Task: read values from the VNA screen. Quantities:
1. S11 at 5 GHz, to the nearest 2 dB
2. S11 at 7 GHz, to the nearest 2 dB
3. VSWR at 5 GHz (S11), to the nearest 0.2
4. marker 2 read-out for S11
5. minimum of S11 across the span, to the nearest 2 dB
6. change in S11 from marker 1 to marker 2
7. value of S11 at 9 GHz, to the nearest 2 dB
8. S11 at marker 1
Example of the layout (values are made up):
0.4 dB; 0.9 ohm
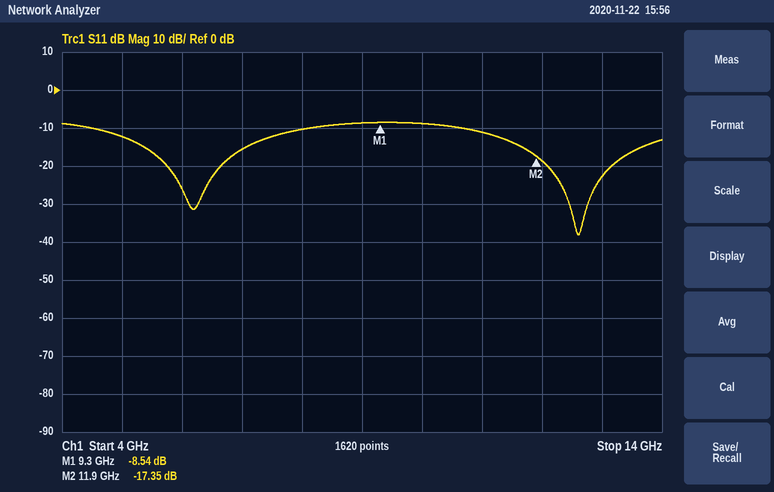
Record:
-12 dB; -16 dB; 1.6; -17.35 dB; -38 dB; -8.81 dB; -8 dB; -8.54 dB
